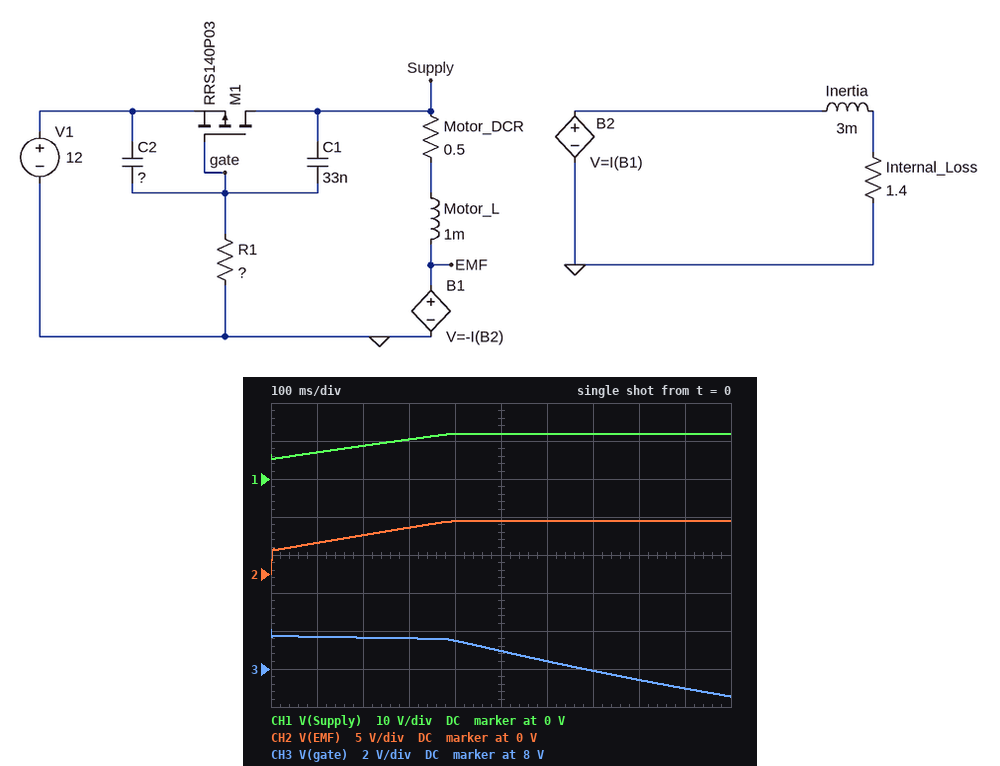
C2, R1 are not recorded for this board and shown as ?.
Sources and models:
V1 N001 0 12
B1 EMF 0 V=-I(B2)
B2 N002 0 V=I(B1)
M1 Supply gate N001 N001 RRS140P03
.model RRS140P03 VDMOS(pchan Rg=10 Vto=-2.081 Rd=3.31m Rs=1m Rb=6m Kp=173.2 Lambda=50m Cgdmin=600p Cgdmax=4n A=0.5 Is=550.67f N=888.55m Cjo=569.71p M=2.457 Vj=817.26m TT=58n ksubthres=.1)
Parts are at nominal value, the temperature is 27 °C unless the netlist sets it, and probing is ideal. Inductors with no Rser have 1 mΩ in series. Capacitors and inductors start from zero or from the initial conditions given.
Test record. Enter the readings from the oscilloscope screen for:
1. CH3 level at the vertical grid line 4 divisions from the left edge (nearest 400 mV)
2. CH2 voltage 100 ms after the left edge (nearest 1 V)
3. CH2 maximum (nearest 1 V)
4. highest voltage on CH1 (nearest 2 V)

9.6 V
4 V
7 V
12 V
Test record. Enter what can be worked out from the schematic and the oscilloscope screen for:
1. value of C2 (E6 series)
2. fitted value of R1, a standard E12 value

68 nF
15 MΩ
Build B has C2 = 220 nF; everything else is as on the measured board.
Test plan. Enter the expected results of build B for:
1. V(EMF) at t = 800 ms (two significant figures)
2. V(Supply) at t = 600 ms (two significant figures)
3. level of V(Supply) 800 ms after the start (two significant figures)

5.7 V
6.6 V
9.7 V
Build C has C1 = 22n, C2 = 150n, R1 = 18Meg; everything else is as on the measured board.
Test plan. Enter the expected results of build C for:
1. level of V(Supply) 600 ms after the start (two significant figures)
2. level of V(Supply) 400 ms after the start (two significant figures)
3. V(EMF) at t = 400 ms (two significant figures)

8.7 V
4.8 V
2.8 V
